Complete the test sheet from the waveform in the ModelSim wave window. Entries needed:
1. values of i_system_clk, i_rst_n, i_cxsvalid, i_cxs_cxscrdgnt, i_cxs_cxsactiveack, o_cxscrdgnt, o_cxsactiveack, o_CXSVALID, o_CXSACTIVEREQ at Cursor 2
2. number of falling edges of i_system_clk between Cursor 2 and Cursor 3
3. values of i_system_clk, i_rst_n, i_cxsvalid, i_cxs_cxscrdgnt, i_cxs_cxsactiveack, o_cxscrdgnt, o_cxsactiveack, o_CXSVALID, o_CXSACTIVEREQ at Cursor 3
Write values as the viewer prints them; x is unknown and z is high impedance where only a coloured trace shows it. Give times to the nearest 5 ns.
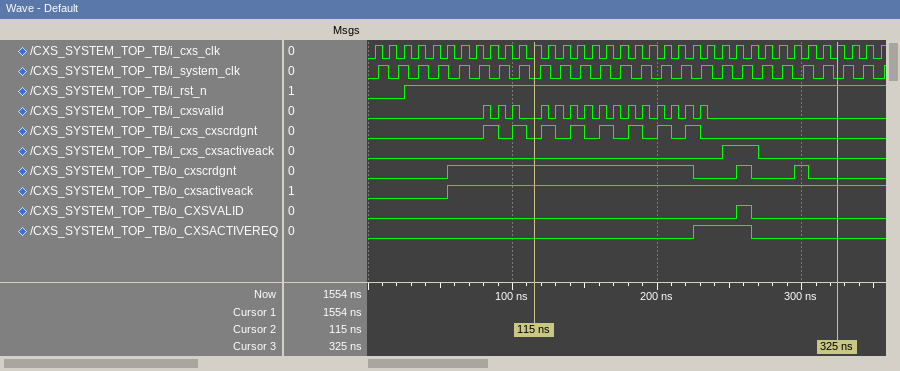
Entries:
i_system_clk=0, i_rst_n=1, i_cxsvalid=0, i_cxs_cxscrdgnt=0, i_cxs_cxsactiveack=0, o_cxscrdgnt=1, o_cxsactiveack=1, o_CXSVALID=0, o_CXSACTIVEREQ=0
15
i_system_clk=0, i_rst_n=1, i_cxsvalid=0, i_cxs_cxscrdgnt=0, i_cxs_cxsactiveack=0, o_cxscrdgnt=0, o_cxsactiveack=1, o_CXSVALID=0, o_CXSACTIVEREQ=0
